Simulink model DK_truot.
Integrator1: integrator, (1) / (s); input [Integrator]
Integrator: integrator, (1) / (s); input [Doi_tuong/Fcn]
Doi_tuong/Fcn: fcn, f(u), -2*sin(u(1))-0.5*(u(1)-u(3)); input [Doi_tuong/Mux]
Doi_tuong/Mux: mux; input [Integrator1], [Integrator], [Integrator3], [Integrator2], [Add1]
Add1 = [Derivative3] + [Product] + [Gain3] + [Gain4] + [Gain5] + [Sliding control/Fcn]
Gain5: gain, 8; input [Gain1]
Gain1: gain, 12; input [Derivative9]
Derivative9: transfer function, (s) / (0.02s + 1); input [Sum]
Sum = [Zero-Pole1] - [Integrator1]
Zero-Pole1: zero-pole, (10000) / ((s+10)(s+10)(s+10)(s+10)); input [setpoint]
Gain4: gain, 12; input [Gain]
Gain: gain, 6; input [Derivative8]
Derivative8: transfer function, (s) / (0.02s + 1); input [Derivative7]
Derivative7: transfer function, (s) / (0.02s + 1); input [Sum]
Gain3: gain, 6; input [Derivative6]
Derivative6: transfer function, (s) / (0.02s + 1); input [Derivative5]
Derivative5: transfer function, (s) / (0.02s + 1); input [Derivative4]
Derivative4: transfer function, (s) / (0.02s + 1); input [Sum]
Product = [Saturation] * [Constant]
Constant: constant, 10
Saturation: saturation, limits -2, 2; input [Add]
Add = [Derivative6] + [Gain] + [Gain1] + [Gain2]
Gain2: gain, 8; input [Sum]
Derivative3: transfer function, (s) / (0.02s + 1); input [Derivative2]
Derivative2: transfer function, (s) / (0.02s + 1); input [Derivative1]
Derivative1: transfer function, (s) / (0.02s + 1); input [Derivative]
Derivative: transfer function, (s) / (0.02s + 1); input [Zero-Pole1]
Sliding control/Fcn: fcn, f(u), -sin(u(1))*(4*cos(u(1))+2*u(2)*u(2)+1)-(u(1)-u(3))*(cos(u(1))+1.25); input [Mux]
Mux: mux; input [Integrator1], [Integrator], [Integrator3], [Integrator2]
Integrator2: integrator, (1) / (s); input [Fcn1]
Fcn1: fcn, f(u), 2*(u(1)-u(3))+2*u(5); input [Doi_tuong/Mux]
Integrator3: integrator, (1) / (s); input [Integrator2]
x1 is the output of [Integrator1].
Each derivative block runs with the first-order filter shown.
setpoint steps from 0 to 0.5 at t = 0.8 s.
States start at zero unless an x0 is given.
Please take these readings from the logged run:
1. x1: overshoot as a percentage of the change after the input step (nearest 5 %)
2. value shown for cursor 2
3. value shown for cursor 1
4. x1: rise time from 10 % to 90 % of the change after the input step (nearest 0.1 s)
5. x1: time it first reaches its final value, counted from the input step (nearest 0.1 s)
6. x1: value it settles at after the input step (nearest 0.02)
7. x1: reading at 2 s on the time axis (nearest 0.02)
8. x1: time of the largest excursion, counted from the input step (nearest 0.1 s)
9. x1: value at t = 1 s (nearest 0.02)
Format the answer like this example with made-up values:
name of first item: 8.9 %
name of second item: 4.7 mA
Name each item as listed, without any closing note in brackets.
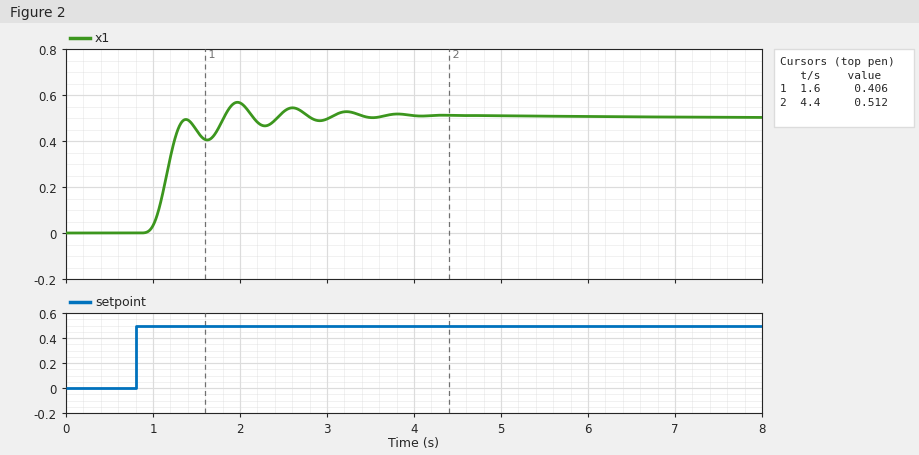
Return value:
x1: overshoot as a percentage of the change after the input step: 15 %
value shown for cursor 2: 0.512
value shown for cursor 1: 0.406
x1: rise time from 10 % to 90 % of the change after the input step: 0.3 s
x1: time it first reaches its final value, counted from the input step: 1.0 s
x1: value it settles at after the input step: 0.50
x1: reading at 2 s on the time axis: 0.56
x1: time of the largest excursion, counted from the input step: 1.2 s
x1: value at t = 1 s: 0.04
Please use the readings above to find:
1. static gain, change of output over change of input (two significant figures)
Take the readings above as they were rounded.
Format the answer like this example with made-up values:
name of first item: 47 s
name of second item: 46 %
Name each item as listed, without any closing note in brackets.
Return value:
static gain, change of output over change of input: 1.0
